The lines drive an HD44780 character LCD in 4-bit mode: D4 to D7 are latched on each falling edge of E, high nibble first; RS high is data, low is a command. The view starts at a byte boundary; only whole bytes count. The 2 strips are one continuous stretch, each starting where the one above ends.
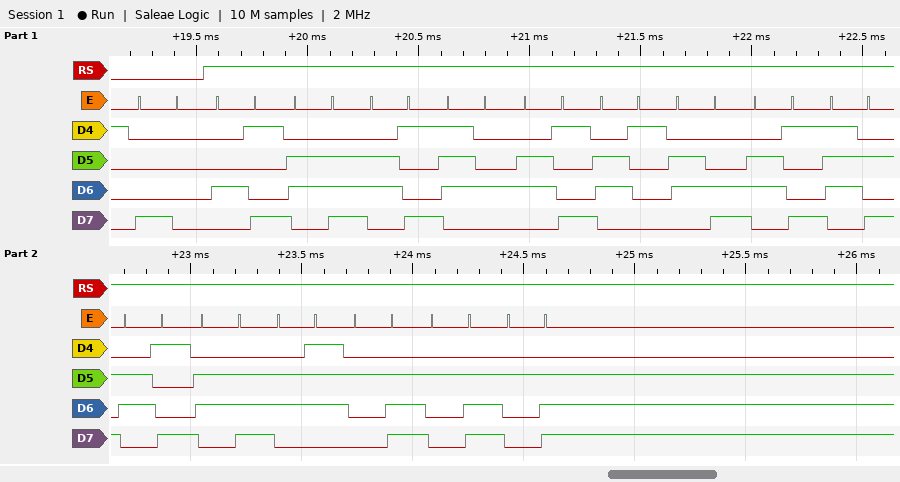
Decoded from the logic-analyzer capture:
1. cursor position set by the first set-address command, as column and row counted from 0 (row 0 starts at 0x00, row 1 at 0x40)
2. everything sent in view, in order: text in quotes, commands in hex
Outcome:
column 0, row 0
0x80 "Initializing..."
